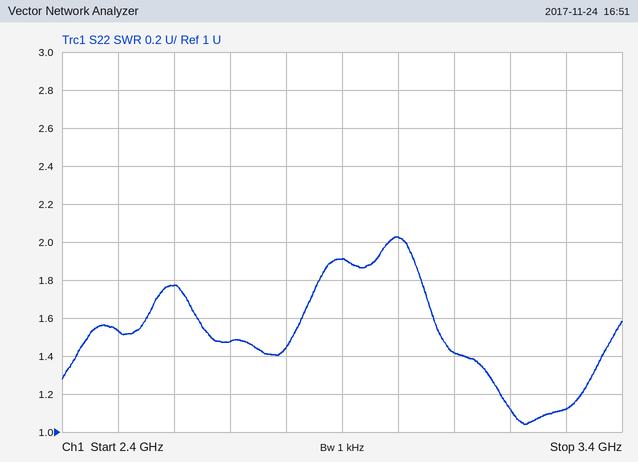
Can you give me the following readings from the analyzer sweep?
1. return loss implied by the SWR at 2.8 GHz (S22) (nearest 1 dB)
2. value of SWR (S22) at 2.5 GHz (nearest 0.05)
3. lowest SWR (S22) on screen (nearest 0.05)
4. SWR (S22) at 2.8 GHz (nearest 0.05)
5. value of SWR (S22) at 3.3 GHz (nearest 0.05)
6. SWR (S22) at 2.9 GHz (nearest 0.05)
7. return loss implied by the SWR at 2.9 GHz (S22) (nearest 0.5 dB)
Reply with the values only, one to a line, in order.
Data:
15 dB
1.55
1.05
1.45
1.10
1.90
10.0 dB
